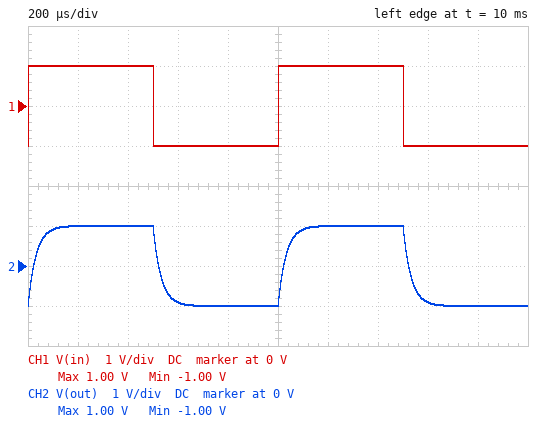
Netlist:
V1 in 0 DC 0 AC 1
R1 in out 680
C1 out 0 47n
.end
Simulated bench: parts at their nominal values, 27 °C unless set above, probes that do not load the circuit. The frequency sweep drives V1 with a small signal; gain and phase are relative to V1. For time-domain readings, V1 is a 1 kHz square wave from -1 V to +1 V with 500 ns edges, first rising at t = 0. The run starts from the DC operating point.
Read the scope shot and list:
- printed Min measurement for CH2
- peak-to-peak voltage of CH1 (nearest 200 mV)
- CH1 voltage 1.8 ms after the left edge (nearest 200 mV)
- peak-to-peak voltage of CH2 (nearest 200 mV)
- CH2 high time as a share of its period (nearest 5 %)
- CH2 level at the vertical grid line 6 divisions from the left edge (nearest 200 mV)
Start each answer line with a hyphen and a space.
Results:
- -1.00 V
- 2.0 V
- -1.0 V
- 2.0 V
- 50 %
- 1.0 V
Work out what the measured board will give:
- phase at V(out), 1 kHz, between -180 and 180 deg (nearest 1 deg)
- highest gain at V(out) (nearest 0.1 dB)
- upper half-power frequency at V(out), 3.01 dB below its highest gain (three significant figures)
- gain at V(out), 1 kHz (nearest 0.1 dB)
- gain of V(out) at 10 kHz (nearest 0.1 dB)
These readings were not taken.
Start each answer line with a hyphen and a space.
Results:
- -11 deg
- 0 dB
- 4.98 kHz
- -0.2 dB
- -7.0 dB
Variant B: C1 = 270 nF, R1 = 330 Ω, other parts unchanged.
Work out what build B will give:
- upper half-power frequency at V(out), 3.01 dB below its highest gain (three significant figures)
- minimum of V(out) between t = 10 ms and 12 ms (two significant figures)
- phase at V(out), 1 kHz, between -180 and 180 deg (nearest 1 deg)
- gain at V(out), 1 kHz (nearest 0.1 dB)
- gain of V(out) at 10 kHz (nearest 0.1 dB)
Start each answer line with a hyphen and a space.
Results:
- 1.79 kHz
- -990 mV
- -29 deg
- -1.2 dB
- -15.1 dB
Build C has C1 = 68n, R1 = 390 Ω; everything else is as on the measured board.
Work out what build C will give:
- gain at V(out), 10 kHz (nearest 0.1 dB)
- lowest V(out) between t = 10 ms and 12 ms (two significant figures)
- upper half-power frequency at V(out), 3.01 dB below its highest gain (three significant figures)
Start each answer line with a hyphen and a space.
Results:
- -5.8 dB
- -1.0 V
- 6.00 kHz
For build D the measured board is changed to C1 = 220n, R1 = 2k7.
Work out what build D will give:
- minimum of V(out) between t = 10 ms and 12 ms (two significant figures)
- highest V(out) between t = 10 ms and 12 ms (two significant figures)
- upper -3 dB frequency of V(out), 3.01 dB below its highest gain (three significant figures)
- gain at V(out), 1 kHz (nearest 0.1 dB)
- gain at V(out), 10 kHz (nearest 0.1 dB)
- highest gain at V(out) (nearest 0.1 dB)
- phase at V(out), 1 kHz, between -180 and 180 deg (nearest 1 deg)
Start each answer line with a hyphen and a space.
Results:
- -400 mV
- 400 mV
- 268 Hz
- -11.7 dB
- -31.4 dB
- 0 dB
- -75 deg
